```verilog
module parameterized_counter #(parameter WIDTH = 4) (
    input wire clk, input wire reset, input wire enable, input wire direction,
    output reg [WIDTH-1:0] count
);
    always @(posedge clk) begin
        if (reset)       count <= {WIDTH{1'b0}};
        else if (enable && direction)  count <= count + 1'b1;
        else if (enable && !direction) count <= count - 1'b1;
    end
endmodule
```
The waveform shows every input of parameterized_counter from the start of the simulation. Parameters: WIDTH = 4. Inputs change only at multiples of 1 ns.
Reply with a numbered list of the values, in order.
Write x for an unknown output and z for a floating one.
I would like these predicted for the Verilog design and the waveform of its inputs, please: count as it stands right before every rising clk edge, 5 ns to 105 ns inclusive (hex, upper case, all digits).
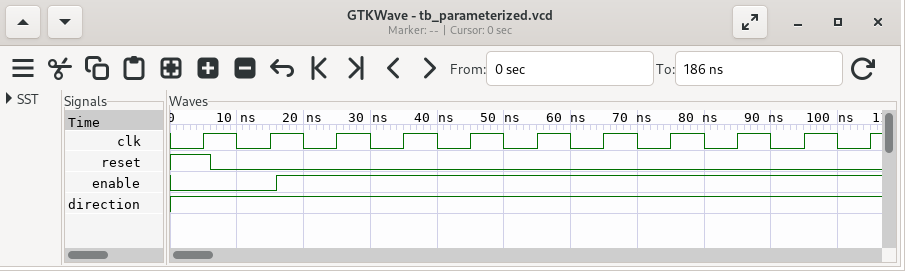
1. x, 0, 0, 1, 2, 3, 4, 5, 6, 7, 8
